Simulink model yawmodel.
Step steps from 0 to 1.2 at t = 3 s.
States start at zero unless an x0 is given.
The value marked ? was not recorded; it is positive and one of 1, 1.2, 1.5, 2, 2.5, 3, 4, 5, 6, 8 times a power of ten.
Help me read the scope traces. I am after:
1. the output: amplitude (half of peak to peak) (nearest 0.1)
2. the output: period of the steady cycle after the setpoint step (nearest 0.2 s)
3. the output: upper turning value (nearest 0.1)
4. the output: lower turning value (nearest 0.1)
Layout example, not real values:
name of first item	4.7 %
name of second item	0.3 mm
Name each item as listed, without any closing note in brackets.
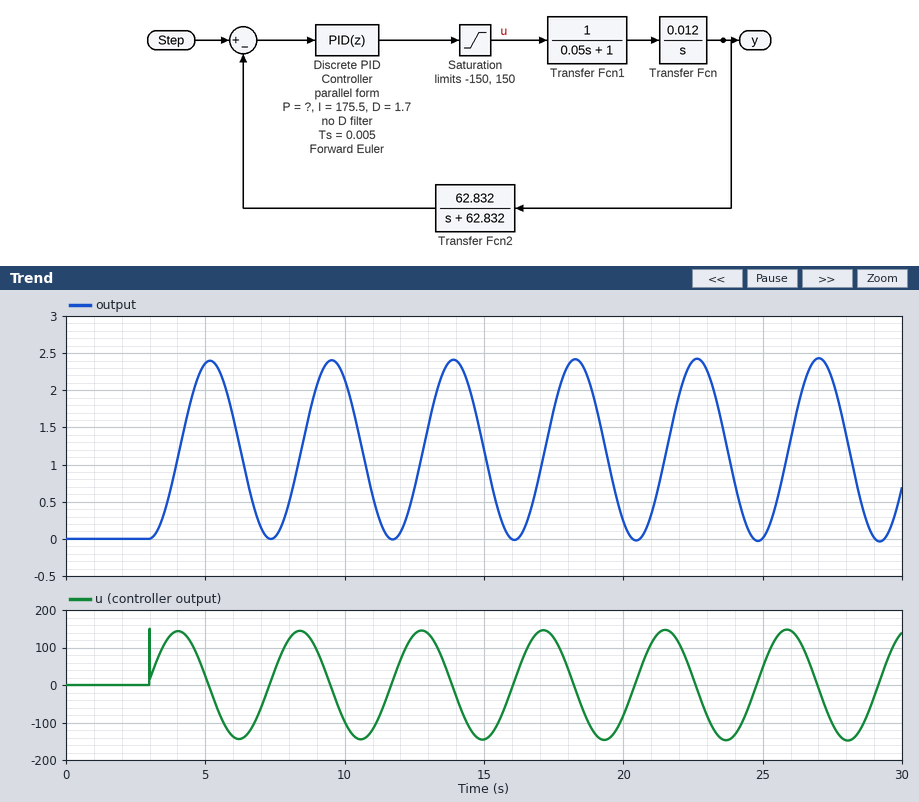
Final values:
the output: amplitude (half of peak to peak)	1.2
the output: period of the steady cycle after the setpoint step	4.4 s
the output: upper turning value	2.4
the output: lower turning value	0.0
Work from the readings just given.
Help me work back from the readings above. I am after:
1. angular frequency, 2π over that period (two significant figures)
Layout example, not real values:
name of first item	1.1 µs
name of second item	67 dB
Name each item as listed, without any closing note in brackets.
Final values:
angular frequency, 2π over that period	1.4 rad/s
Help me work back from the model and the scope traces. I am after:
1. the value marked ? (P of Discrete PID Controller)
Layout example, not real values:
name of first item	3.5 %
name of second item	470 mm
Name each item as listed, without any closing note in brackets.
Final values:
the value marked ?	12
